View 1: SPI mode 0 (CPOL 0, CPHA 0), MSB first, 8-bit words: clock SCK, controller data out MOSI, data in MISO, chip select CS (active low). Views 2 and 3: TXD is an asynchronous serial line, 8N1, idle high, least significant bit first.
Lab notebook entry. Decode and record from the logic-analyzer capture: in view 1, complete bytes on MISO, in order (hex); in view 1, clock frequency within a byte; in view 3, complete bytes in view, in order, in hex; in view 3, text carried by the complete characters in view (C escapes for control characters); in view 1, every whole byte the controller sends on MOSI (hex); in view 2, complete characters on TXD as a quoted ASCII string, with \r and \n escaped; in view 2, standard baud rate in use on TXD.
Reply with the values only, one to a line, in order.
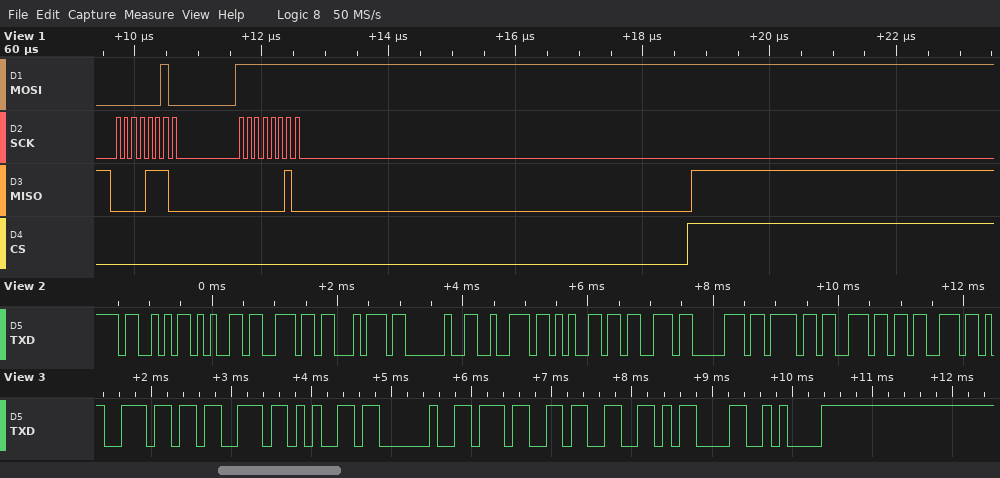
0x0E 0x02
8 MHz
6E 73 65 20 37 33 0D 0A
"nse 73\r\n"
0x02 0xFF
"Sent respons"
9600 baud
